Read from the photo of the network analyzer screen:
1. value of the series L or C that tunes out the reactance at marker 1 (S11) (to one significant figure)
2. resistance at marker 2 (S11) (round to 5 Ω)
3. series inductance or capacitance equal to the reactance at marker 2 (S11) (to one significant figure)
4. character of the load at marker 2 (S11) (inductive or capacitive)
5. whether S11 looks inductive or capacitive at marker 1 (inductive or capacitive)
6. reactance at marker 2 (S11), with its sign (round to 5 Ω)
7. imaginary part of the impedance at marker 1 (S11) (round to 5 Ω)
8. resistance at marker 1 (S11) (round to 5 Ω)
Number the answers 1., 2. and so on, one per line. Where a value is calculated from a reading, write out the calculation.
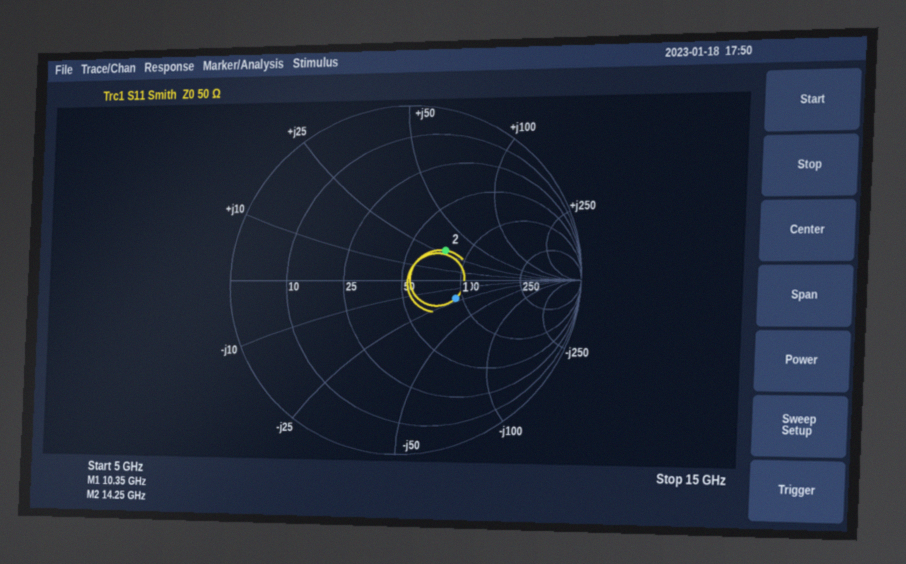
1. L = 20 Ω/(2π × 10.35 GHz) ≈ 308 pH, so 300 pH to one significant figure
2. 75 Ω
3. L = 30 Ω/(2π × 14.25 GHz) ≈ 335 pH, so 300 pH to one significant figure
4. inductive
5. capacitive
6. +30 Ω
7. -20 Ω
8. 90 Ω
